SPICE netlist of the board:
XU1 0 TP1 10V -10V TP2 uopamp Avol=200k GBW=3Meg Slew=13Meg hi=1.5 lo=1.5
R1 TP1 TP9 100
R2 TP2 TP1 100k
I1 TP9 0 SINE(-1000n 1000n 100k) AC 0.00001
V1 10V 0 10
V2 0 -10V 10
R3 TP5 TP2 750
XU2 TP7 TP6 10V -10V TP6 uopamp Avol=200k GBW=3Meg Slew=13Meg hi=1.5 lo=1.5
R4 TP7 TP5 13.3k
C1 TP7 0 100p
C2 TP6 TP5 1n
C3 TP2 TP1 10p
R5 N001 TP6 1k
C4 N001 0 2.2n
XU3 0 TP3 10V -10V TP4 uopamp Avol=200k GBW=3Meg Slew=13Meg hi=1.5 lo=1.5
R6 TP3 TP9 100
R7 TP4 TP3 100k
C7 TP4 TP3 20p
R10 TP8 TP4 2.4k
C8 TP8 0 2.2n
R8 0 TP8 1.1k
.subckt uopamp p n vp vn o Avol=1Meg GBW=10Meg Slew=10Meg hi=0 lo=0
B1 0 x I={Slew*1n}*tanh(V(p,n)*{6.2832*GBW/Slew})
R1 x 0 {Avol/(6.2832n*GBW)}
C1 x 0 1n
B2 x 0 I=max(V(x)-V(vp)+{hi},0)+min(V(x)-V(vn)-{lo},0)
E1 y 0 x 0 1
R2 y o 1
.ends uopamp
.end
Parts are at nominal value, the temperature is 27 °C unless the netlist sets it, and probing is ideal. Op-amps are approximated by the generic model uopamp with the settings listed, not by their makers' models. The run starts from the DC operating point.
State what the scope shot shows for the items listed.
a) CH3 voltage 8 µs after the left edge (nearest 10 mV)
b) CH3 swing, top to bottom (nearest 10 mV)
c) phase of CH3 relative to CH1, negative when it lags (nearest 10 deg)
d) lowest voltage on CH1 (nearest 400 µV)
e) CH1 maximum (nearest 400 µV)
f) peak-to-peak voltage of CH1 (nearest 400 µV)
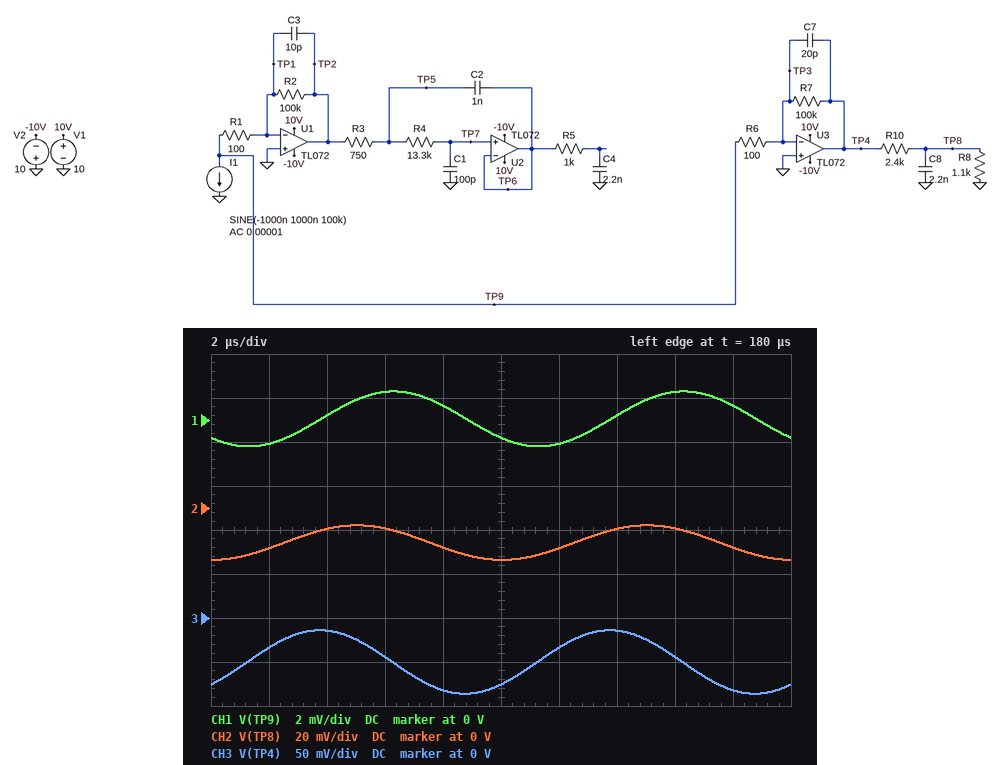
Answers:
-80 mV
70 mV
90 deg
-1.2 mV
1.2 mV
2.4 mV
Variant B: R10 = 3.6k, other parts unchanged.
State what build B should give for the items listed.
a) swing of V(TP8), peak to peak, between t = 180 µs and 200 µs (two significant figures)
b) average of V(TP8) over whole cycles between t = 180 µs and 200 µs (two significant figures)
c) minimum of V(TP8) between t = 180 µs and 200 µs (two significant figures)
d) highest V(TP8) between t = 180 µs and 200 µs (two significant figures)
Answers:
11 mV
-12 mV
-17 mV
-6.2 mV
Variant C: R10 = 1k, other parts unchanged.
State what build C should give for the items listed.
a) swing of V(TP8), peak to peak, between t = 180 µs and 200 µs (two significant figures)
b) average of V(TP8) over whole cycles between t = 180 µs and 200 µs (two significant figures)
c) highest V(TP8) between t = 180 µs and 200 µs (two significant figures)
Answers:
31 mV
-26 mV
-11 mV
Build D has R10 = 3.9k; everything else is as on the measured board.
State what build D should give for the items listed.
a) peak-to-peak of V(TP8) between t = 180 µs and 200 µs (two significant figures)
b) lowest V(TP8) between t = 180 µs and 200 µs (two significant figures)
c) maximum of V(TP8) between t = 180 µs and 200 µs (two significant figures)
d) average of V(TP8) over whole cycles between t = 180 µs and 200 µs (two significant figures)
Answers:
10 mV
-16 mV
-5.9 mV
-11 mV
